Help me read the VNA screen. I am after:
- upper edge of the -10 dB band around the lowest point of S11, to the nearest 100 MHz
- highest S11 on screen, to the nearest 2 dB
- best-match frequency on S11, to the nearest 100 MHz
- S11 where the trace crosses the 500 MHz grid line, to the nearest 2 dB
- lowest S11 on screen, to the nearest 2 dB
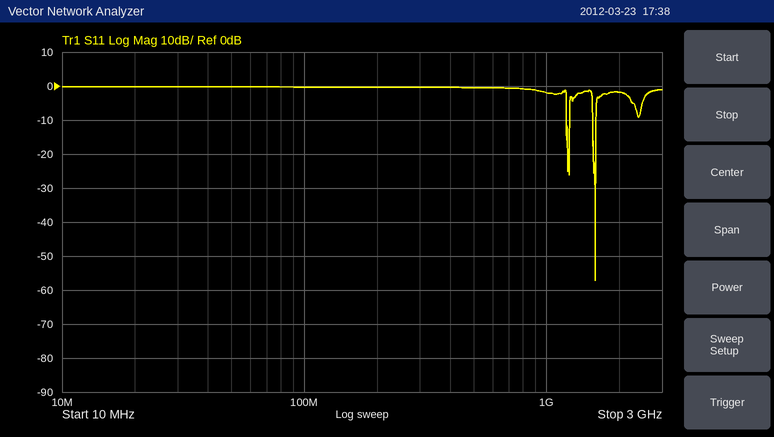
1.6 GHz
0 dB
1.6 GHz
0 dB
-58 dB
